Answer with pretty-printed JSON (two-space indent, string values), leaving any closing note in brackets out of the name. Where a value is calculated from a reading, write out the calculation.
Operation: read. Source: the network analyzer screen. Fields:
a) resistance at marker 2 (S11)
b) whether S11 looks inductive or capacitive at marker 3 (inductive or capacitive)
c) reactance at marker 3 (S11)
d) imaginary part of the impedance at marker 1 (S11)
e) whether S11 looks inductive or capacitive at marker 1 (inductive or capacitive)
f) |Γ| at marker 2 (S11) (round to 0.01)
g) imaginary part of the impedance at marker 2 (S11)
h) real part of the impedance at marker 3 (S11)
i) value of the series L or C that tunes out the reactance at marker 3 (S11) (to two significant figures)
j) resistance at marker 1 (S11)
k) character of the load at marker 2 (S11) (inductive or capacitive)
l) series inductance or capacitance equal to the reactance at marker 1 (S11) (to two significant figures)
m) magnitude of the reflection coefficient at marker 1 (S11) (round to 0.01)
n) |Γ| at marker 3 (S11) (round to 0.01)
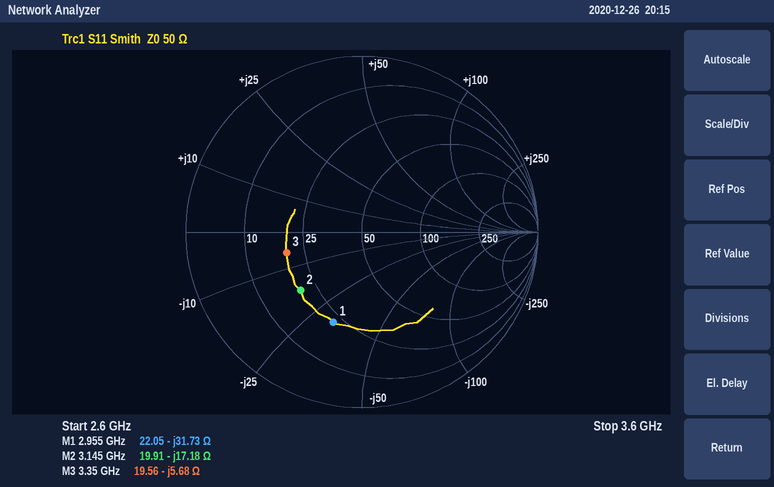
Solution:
{
  "resistance at marker 2": "19.91 Ω",
  "whether S11 looks inductive or capacitive at marker 3": "capacitive",
  "reactance at marker 3": "-5.68 Ω",
  "imaginary part of the impedance at marker 1": "-31.73 Ω",
  "whether S11 looks inductive or capacitive at marker 1": "capacitive",
  "|Γ| at marker 2 (S11)": "0.48",
  "imaginary part of the impedance at marker 2": "-17.18 Ω",
  "real part of the impedance at marker 3": "19.56 Ω",
  "value of the series L or C that tunes out the reactance at marker 3 (S11)": "L = 5.68 Ω/(2π × 3.35 GHz) ≈ 270 pH",
  "resistance at marker 1": "22.05 Ω",
  "character of the load at marker 2 (S11)": "capacitive",
  "series inductance or capacitance equal to the reactance at marker 1 (S11)": "C = 1/(2π × 2.955 GHz × 31.73 Ω) ≈ 1.7 pF",
  "magnitude of the reflection coefficient at marker 1 (S11)": "0.54",
  "|Γ| at marker 3 (S11)": "0.44"
}
